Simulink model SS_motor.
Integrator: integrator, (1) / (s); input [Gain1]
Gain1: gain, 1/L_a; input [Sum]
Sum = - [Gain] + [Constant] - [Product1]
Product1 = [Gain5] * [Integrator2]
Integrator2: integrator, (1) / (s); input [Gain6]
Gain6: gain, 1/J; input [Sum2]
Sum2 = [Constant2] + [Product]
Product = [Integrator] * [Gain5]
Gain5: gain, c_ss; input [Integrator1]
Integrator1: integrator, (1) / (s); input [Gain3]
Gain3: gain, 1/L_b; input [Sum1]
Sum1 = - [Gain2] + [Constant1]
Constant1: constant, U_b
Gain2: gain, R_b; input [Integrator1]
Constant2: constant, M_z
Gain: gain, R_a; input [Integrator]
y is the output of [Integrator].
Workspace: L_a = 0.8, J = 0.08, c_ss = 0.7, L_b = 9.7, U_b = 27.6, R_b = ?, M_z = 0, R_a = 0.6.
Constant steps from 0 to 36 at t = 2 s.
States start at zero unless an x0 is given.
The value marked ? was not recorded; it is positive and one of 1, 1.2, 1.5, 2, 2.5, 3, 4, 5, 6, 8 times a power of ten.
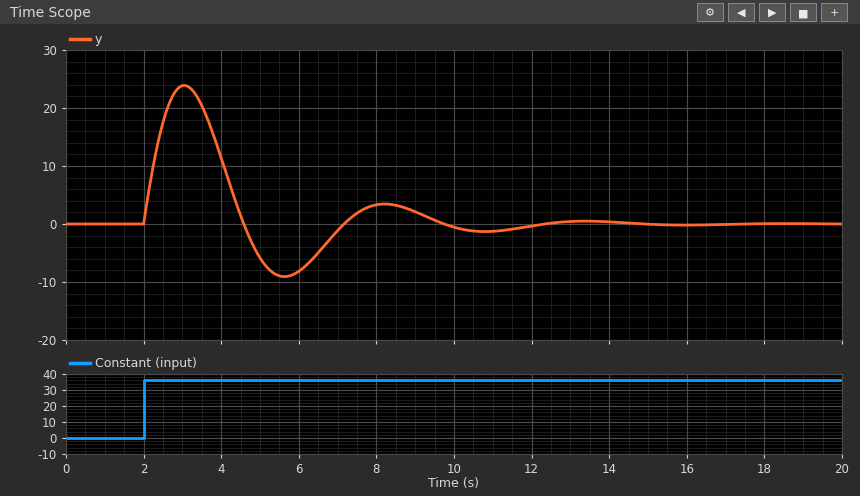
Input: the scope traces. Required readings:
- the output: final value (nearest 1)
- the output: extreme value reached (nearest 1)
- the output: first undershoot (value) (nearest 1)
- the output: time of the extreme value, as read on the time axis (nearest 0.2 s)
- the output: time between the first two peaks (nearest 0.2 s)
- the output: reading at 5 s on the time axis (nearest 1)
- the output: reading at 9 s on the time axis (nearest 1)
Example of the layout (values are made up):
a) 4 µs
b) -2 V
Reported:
a) 0
b) 24
c) -9
d) 3.0 s
e) 5.2 s
f) -6
g) 2
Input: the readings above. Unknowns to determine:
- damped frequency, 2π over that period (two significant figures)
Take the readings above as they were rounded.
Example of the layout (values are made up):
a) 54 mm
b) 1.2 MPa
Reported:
a) 1.2 rad/s
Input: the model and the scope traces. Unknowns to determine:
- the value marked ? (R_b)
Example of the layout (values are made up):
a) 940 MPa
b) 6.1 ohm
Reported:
a) 60
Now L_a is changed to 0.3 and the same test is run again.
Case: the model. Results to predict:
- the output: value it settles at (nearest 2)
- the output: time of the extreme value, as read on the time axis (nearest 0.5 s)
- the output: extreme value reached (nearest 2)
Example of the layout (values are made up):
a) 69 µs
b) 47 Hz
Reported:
a) 0
b) 2.5 s
c) 32
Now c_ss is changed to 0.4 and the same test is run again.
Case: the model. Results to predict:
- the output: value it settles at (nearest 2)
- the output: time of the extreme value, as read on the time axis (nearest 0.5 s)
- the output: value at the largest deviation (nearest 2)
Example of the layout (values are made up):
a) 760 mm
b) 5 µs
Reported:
a) 0
b) 3.5 s
c) 34
